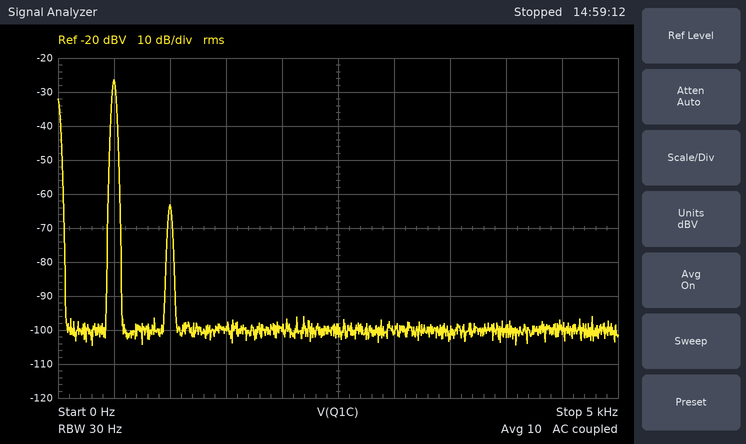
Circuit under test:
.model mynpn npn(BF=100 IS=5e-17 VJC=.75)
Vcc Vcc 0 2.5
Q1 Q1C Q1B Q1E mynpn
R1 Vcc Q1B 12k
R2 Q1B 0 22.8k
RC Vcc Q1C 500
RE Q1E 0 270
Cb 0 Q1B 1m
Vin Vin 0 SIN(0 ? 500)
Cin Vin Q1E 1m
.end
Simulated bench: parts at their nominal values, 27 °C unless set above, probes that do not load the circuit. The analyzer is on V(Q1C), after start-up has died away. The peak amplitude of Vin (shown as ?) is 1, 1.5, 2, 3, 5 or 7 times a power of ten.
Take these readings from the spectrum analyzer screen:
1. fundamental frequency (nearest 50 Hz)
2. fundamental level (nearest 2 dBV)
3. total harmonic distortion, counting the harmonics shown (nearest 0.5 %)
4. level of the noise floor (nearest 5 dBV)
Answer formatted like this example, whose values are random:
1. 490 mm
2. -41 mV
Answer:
1. 500 Hz
2. -26 dBV
3. 1.5 %
4. -100 dBV
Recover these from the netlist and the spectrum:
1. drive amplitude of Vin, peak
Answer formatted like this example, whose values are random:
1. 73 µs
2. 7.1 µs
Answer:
1. 1.5 mV
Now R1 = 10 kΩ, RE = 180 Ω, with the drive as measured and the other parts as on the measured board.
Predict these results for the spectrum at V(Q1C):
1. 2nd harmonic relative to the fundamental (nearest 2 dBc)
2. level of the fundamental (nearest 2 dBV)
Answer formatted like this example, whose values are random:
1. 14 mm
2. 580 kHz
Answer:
1. -18 dBc
2. -26 dBV
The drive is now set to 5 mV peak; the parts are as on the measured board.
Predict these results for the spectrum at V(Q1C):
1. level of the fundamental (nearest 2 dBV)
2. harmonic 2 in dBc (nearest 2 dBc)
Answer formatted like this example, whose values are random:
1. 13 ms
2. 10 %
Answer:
1. -16 dBV
2. -26 dBc
